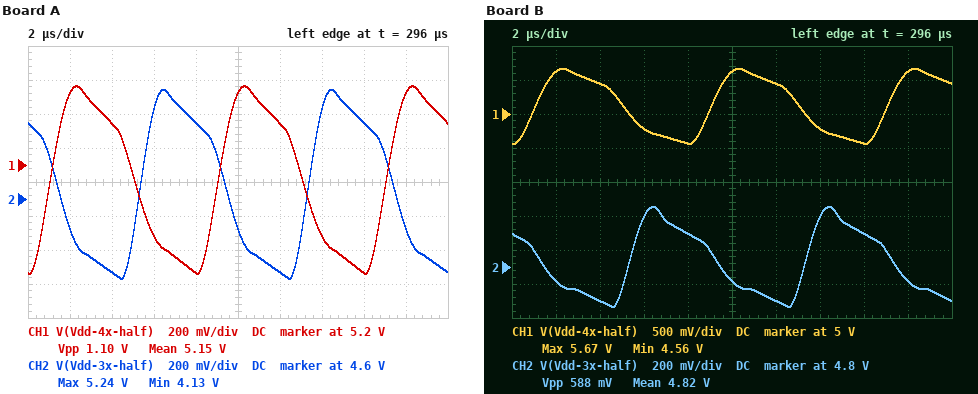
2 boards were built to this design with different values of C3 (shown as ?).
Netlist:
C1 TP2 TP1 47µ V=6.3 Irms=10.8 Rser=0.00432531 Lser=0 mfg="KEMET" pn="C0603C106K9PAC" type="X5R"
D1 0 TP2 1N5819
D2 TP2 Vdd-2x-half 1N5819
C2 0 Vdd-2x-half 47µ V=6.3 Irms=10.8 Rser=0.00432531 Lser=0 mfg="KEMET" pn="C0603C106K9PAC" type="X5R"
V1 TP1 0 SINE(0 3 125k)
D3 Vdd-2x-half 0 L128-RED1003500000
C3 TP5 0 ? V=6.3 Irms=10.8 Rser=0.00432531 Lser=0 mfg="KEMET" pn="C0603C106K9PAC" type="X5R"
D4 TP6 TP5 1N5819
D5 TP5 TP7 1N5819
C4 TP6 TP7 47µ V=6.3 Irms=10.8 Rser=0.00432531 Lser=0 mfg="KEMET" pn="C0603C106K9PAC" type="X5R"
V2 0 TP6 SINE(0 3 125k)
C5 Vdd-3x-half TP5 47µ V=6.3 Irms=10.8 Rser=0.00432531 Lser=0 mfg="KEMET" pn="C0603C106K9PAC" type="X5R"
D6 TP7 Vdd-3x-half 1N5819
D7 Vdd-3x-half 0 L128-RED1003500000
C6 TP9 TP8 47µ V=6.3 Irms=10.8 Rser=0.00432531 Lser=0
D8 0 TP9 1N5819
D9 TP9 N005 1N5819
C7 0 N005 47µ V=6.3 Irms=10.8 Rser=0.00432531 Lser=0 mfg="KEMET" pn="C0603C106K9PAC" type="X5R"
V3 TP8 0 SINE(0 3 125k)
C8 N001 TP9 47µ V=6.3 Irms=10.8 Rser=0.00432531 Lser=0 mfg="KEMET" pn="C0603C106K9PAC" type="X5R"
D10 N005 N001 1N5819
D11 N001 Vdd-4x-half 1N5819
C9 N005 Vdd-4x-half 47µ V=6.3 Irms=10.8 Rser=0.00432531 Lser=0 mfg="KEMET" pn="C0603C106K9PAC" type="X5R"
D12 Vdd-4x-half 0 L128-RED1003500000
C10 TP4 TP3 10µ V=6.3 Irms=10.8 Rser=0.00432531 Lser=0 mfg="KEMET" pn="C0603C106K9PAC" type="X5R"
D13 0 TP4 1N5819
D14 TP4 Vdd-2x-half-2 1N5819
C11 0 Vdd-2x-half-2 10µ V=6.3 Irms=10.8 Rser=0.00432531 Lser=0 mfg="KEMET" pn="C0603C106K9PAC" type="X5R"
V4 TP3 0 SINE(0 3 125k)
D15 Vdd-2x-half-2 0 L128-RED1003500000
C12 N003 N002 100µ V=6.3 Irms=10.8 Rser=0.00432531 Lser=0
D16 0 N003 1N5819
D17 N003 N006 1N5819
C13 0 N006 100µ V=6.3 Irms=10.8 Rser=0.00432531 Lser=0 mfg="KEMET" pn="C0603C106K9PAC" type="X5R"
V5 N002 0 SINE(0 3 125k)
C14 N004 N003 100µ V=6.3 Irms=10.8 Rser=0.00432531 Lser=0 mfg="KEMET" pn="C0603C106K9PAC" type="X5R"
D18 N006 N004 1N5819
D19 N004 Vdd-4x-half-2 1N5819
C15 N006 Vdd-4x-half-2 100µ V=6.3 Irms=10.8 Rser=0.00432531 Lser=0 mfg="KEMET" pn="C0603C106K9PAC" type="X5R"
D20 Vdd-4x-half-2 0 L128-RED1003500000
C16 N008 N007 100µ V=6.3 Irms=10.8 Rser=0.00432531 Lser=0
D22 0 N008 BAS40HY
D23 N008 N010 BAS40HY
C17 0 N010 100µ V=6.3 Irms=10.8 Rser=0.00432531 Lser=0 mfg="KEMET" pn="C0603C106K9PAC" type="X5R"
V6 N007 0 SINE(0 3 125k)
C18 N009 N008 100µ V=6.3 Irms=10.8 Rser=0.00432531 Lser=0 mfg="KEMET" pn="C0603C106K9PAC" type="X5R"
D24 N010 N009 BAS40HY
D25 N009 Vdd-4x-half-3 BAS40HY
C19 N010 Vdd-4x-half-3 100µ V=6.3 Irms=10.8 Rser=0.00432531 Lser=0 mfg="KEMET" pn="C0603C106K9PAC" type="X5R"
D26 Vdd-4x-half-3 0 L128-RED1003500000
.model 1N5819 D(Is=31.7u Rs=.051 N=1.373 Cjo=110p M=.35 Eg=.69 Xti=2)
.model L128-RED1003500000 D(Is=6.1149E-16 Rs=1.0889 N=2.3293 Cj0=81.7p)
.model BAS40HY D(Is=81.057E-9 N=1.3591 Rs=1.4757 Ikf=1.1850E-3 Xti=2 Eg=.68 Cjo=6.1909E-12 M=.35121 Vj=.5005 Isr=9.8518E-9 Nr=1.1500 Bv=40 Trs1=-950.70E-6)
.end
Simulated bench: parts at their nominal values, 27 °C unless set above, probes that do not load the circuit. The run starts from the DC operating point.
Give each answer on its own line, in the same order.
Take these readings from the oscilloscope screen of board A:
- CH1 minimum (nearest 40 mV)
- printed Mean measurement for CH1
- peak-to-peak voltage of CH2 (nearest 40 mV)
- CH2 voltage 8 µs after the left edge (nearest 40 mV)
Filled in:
4.56 V
5.15 V
1.12 V
5.04 V
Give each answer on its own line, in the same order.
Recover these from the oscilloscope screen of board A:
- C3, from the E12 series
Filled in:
39 µF
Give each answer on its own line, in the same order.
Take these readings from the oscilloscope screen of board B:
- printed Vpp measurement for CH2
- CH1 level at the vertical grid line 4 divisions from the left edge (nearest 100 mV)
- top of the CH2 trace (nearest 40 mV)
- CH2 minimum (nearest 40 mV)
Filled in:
588 mV
4.6 V
5.16 V
4.56 V
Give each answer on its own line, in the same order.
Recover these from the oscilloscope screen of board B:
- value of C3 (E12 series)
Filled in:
150 µF
